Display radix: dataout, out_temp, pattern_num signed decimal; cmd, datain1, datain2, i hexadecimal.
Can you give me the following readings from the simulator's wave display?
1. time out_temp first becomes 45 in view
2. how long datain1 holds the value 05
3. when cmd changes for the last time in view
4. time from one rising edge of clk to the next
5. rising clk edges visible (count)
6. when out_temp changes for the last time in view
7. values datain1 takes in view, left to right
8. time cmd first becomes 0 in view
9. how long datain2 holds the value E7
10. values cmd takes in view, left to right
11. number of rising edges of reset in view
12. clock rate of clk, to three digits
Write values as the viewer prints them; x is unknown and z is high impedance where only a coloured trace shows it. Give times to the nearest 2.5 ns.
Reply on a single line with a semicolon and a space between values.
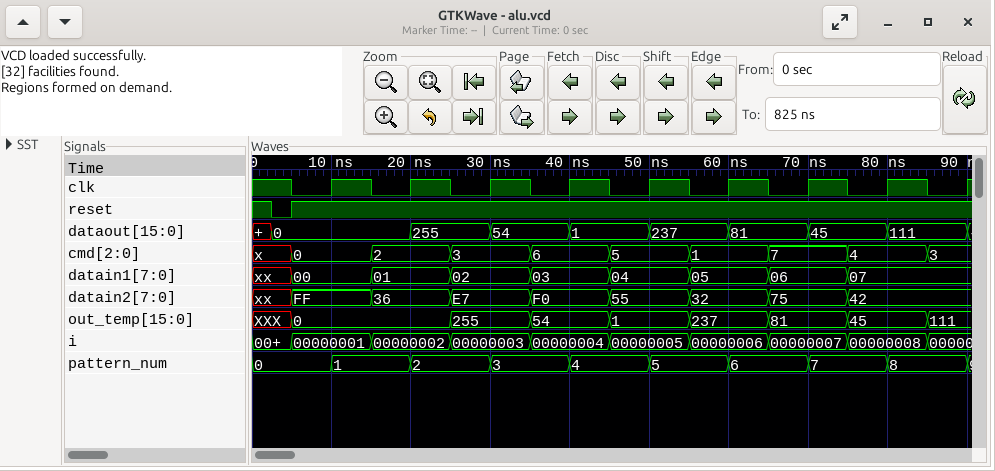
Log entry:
75 ns; 10 ns; 85 ns; 10 ns; 9; 85 ns; xx, 00, 01, 02, 03, 04, 05, 06, 07; 5 ns; 10 ns; x, 0, 2, 3, 6, 5, 1, 7, 4, 3; 1; 100 MHz
